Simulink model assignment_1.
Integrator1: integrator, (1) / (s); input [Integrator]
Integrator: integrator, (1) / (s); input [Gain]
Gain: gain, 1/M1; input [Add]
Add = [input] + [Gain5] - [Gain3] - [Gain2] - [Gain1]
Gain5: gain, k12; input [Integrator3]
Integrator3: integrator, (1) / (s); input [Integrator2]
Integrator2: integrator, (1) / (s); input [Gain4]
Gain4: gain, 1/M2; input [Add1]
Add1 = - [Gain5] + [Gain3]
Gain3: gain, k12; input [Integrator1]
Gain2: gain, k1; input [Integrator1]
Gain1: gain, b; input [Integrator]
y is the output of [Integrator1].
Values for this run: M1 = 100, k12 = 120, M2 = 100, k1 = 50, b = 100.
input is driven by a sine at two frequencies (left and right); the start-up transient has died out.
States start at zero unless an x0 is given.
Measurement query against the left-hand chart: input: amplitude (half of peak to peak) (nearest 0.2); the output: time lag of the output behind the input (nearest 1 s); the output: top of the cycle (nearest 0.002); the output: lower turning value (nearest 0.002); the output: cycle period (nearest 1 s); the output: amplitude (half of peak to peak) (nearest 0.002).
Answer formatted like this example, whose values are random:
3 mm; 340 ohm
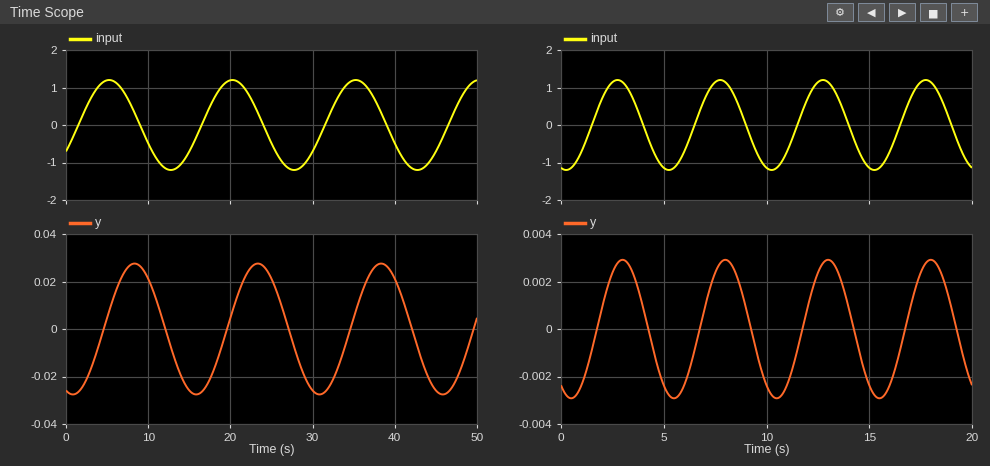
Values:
1.2; 3 s; 0.028; -0.028; 15 s; 0.028
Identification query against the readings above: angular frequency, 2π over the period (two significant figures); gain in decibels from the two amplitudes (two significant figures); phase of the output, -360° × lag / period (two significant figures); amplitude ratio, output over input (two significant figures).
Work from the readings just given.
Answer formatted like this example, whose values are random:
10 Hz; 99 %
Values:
0.42 rad/s; -33 dB; -72°; 0.023
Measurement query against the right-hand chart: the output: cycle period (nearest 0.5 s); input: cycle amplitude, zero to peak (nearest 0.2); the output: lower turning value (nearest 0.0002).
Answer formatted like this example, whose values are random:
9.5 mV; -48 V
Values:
5.0 s; 1.2; -0.0030
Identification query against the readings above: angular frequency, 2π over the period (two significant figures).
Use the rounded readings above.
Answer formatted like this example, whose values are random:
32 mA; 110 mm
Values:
1.3 rad/s
